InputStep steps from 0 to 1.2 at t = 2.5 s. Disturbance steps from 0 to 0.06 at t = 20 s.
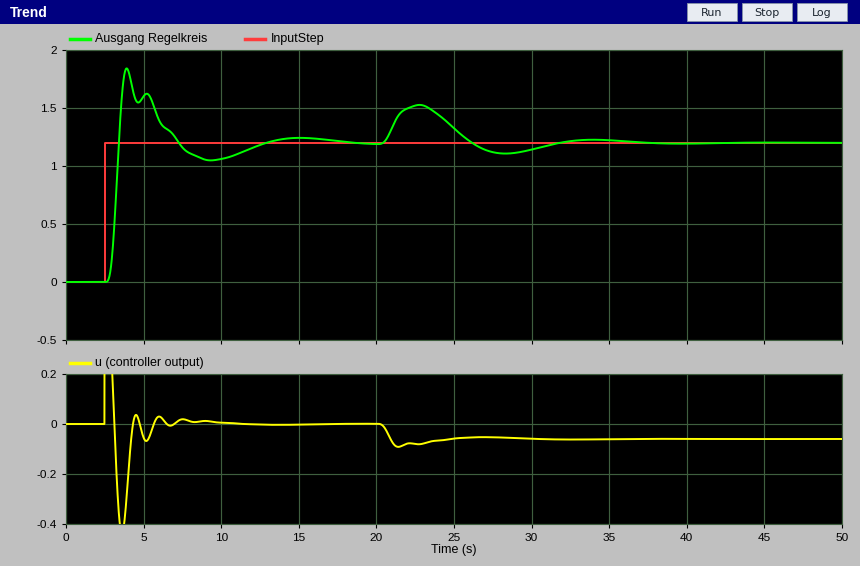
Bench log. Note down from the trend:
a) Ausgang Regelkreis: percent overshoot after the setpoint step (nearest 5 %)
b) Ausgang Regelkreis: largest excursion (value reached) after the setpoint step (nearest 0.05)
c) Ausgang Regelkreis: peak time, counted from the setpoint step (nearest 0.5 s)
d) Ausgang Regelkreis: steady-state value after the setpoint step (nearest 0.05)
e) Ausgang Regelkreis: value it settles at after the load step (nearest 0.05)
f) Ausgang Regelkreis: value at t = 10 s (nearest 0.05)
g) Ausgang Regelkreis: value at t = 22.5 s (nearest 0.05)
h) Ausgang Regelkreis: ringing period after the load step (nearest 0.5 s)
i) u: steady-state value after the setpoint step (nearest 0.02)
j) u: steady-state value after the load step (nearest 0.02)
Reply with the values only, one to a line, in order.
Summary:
55 %
1.85
1.5 s
1.20
1.20
1.05
1.50
11.0 s
0.00
-0.06
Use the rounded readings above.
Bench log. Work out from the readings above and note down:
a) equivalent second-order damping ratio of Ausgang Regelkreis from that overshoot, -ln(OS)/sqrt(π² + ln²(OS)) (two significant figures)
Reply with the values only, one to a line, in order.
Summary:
0.19
